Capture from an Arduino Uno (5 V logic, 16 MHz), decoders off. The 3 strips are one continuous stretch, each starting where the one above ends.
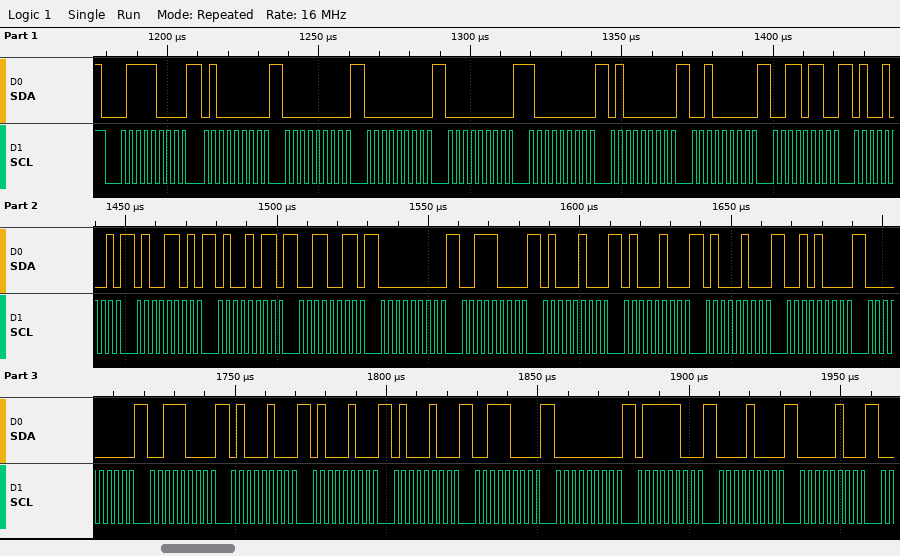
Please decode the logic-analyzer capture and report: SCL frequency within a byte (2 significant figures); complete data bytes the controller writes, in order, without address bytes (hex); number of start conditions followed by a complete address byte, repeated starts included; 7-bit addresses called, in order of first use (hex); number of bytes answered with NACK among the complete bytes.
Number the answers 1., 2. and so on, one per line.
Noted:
1. 400 kHz
2. 40 00 00 00 80 40 20 36 49 4D 4B 33 00 38 44 44 44 28 00 38 44 44 44 38 00 7C 08 04
3. 1
4. 0x3C
5. 0
